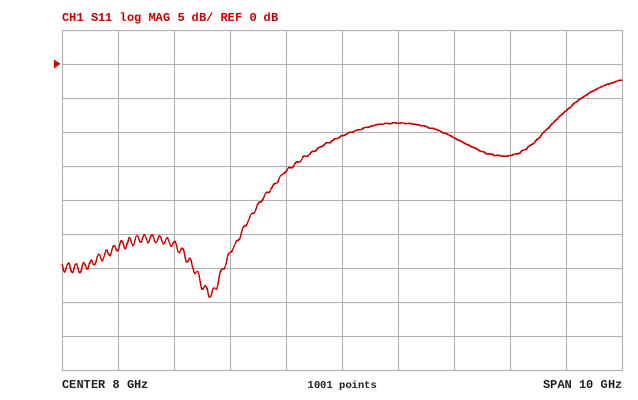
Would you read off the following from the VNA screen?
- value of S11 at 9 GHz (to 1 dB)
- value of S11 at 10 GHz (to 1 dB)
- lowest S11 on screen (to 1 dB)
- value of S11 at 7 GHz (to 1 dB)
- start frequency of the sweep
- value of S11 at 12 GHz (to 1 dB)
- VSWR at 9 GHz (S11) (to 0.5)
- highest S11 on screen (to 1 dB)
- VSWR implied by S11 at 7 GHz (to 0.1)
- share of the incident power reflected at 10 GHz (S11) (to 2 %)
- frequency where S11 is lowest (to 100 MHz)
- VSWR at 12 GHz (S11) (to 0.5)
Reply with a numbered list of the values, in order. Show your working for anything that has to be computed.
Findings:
1. -9 dB
2. -11 dB
3. -34 dB
4. -16 dB
5. 3 GHz
6. -7 dB
7. |Γ| = 10^(-9/20) = 0.3548; VSWR = (1 + 0.3548)/(1 − 0.3548) ≈ 2.10, so 2.0 to the nearest 0.5
8. -2 dB
9. |Γ| = 10^(-16/20) = 0.1585; VSWR = (1 + 0.1585)/(1 − 0.1585) ≈ 1.4
10. 10^(-11/10) ≈ 8 %
11. 5.6 GHz
12. |Γ| = 10^(-7/20) = 0.4467; VSWR = (1 + 0.4467)/(1 − 0.4467) ≈ 2.61, so 2.5 to the nearest 0.5
